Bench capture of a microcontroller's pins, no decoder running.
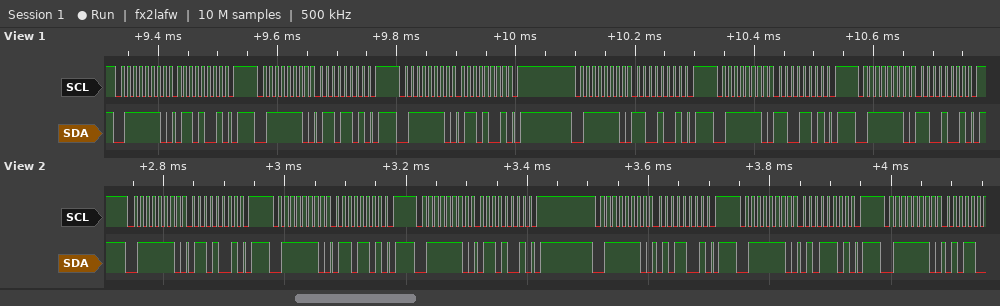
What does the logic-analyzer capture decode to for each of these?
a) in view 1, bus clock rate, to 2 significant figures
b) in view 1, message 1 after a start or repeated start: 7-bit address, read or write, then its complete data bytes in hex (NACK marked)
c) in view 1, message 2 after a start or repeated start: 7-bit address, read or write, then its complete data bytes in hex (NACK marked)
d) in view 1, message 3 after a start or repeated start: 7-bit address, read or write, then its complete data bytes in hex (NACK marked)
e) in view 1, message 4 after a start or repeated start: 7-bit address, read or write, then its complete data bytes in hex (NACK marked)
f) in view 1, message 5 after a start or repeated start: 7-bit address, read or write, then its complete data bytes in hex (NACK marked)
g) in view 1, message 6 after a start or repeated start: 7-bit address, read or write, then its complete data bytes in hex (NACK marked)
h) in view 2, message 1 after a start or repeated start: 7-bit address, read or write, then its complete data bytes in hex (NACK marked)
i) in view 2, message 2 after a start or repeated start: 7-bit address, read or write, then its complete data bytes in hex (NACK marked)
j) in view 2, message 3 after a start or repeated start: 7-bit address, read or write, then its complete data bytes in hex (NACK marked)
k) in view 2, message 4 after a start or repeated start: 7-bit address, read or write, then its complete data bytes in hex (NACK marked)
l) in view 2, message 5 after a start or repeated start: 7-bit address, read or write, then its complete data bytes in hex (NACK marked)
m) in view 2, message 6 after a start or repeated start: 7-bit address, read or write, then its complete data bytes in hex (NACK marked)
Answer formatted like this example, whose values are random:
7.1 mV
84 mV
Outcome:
100 kHz
0x3F write: 69
0x3F write: 6D
0x3F write: 69
0x3F write: C9
0x3F write: CD
0x3F write: C9
0x3F write: 69
0x3F write: 6D
0x3F write: 69
0x3F write: 59
0x3F write: 5D
0x3F write
